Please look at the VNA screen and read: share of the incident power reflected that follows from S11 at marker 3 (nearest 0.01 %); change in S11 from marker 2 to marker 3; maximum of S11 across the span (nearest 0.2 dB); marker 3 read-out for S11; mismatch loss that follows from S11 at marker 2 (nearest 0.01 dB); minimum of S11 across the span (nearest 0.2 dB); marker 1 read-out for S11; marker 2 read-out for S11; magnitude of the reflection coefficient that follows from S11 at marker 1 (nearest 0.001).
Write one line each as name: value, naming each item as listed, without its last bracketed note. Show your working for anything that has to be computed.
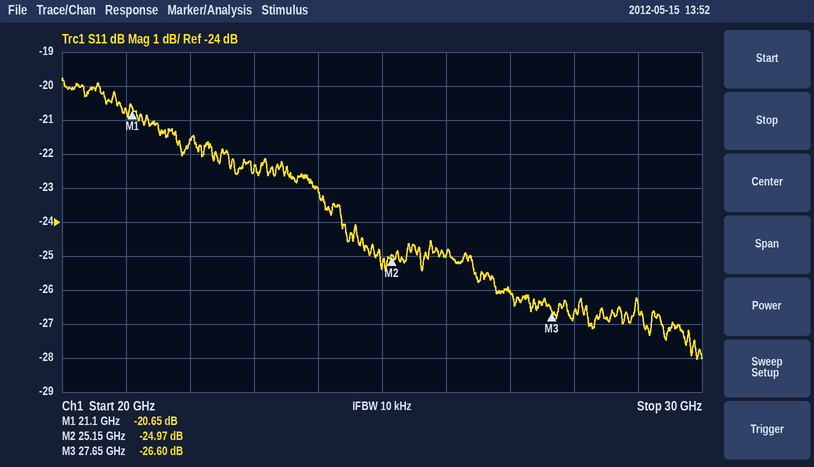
share of the incident power reflected that follows from S11 at marker 3: 10^(-26.6/10) ≈ 0.22 %
change in S11 from marker 2 to marker 3: -26.6 − (-24.97) = -1.63 dB
maximum of S11 across the span: -19.8 dB
marker 3 read-out for S11: -26.60 dB
mismatch loss that follows from S11 at marker 2: −10 log10(1 − 10^(-24.97/10)) ≈ 0.01 dB
minimum of S11 across the span: -28.0 dB
marker 1 read-out for S11: -20.65 dB
marker 2 read-out for S11: -24.97 dB
magnitude of the reflection coefficient that follows from S11 at marker 1: 10^(-20.65/20) ≈ 0.093
